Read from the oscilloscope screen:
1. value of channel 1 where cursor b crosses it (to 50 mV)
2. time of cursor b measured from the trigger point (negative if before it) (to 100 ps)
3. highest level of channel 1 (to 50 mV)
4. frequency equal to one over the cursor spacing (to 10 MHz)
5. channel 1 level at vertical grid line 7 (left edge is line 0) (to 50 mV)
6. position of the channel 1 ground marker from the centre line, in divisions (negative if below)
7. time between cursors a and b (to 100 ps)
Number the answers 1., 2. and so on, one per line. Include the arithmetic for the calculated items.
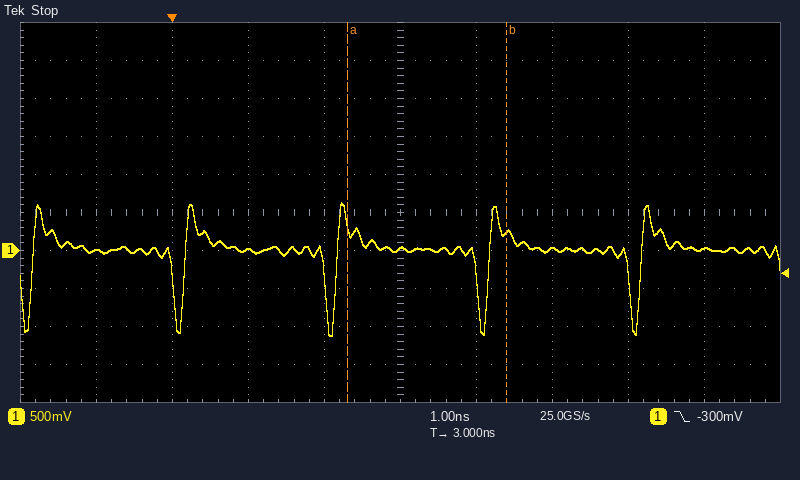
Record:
1. 250 mV
2. +4.4 ns
3. 650 mV
4. 1 / 2.1 ns ≈ 480 MHz
5. 0 mV
6. -1.0 div
7. 2.1 ns
